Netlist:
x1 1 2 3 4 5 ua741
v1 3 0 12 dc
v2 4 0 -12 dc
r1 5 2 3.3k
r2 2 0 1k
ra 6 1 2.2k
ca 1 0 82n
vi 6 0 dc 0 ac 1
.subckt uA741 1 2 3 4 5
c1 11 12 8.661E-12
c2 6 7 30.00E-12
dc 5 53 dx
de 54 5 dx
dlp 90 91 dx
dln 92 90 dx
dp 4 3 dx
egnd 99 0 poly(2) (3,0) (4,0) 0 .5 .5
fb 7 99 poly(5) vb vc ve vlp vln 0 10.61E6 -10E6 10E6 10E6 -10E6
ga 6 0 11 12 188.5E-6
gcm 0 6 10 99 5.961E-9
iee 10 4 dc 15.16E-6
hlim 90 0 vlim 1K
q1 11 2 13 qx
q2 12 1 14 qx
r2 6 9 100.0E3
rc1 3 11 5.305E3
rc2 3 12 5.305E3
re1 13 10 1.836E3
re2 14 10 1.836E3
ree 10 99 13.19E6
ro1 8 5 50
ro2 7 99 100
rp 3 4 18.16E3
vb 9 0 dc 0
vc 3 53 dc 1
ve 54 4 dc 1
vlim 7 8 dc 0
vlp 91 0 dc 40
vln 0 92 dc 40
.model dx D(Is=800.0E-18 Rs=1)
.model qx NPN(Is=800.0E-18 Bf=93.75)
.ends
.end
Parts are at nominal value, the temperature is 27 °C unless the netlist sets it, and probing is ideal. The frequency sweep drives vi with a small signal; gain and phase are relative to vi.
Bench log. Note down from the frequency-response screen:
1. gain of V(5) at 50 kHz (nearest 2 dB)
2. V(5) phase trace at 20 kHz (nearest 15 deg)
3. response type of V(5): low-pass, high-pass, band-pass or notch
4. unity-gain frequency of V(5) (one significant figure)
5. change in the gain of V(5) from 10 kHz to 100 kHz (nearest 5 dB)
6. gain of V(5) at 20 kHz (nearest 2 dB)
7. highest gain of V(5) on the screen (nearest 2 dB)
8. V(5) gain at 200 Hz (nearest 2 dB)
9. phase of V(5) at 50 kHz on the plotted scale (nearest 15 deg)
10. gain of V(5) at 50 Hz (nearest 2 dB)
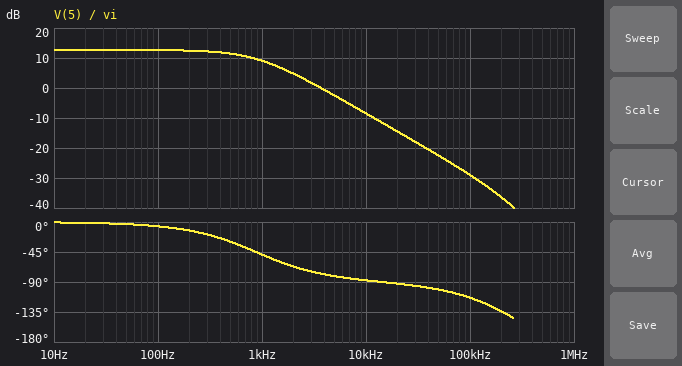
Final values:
-22 dB
-90 deg
low-pass
4 kHz
-20 dB
-14 dB
12 dB
12 dB
-105 deg
12 dB
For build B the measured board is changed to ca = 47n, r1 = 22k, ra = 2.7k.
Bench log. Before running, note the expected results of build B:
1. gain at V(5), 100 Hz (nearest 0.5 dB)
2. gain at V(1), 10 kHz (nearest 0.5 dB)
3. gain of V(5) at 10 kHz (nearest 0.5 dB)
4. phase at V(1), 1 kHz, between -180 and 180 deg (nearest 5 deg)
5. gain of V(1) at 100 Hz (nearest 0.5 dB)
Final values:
27.0 dB
-18.0 dB
9.0 dB
-40 deg
0 dB
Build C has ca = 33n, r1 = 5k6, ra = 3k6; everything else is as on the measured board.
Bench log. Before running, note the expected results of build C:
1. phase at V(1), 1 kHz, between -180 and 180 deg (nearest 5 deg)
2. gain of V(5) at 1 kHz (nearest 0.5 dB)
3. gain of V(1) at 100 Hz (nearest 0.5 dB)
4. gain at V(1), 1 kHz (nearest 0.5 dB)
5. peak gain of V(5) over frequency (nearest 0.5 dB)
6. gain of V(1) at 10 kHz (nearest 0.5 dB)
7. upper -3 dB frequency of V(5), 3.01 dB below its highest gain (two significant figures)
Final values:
-35 deg
14.5 dB
0 dB
-2.0 dB
16.5 dB
-17.5 dB
1.3 kHz
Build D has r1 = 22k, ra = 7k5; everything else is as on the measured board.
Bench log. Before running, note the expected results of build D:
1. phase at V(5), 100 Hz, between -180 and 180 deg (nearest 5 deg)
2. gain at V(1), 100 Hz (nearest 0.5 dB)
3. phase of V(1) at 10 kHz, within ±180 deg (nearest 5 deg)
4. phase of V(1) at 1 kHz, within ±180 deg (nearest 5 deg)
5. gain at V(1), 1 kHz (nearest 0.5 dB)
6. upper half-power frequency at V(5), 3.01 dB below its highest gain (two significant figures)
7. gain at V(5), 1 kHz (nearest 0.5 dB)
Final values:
-20 deg
-0.5 dB
-90 deg
-75 deg
-12.0 dB
260 Hz
15.0 dB
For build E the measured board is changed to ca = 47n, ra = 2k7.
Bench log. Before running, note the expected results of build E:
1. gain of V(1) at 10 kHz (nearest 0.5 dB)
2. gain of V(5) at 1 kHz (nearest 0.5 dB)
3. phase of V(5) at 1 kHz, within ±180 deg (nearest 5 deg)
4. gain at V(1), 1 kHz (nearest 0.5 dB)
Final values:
-18.0 dB
10.5 dB
-40 deg
-2.0 dB
